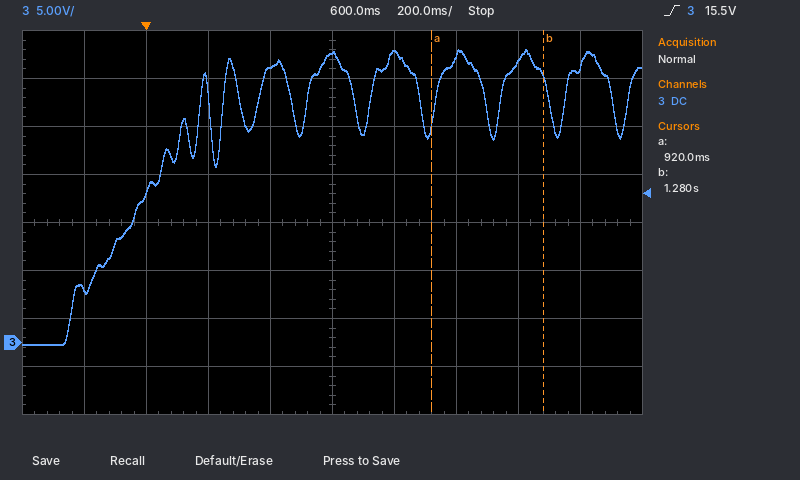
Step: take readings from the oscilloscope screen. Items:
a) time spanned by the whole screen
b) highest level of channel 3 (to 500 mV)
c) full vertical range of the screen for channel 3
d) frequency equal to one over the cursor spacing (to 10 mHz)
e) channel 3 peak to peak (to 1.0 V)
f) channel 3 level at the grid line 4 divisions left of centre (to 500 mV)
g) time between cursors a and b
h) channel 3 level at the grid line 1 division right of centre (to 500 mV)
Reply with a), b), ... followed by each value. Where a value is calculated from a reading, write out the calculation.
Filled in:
a) 2 s
b) 30.5 V
c) 40 V
d) 1 / 360 ms ≈ 2.78 Hz
e) 31.0 V
f) 5.5 V
g) 1.28 s − (920 ms) = 360 ms
h) 30.5 V
